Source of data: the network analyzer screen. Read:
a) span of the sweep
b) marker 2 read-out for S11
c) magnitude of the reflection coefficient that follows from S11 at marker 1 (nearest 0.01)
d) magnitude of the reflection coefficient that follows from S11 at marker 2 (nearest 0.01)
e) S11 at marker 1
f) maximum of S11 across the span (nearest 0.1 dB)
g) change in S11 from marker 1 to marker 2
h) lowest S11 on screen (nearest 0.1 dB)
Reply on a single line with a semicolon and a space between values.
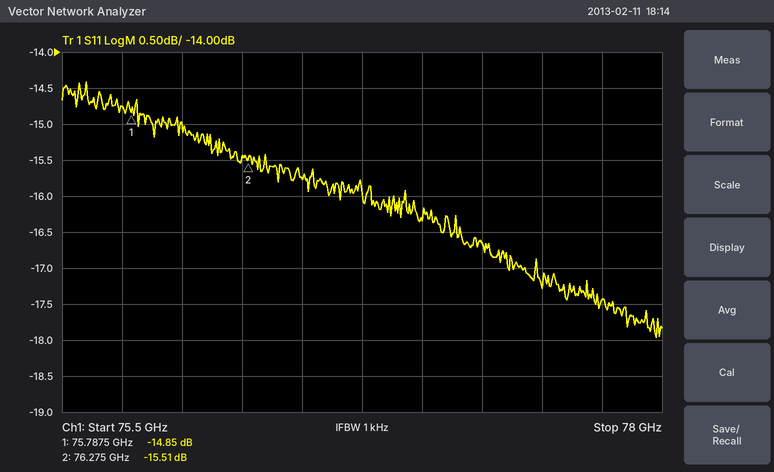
2.5 GHz; -15.51 dB; 0.18; 0.17; -14.85 dB; -14.4 dB; -0.66 dB; -18.0 dB
